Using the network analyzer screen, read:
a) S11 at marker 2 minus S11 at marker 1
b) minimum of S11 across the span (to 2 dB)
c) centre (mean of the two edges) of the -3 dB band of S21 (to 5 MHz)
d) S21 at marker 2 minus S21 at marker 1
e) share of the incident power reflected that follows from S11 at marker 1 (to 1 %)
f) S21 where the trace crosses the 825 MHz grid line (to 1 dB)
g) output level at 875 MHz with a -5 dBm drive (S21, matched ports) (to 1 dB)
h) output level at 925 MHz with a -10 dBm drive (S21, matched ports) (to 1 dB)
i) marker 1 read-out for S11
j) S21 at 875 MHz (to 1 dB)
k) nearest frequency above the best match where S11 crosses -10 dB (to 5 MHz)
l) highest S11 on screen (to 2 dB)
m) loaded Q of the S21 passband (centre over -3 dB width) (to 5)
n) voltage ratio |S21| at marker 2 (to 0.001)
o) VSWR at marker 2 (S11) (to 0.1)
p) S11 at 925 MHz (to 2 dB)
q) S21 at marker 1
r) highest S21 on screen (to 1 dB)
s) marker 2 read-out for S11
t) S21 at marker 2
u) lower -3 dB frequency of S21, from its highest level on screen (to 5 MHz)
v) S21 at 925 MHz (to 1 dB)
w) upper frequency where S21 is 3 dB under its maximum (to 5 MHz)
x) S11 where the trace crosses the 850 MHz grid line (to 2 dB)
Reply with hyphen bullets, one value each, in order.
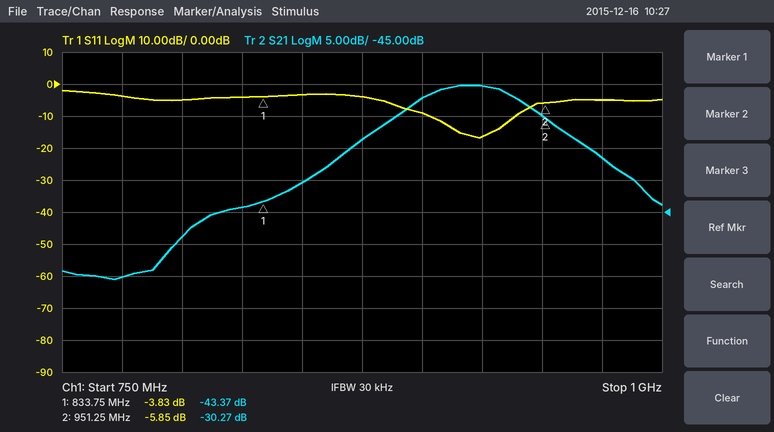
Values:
- -2.02 dB
- -16 dB
- 920 MHz
- 13.10 dB
- 41 %
- -44 dB
- -39 dBm
- -35 dBm
- -3.83 dB
- -34 dB
- 940 MHz
- -2 dB
- 20
- 0.031
- 3.1
- -16 dB
- -43.37 dB
- -25 dB
- -5.85 dB
- -30.27 dB
- 895 MHz
- -25 dB
- 945 MHz
- -4 dB
